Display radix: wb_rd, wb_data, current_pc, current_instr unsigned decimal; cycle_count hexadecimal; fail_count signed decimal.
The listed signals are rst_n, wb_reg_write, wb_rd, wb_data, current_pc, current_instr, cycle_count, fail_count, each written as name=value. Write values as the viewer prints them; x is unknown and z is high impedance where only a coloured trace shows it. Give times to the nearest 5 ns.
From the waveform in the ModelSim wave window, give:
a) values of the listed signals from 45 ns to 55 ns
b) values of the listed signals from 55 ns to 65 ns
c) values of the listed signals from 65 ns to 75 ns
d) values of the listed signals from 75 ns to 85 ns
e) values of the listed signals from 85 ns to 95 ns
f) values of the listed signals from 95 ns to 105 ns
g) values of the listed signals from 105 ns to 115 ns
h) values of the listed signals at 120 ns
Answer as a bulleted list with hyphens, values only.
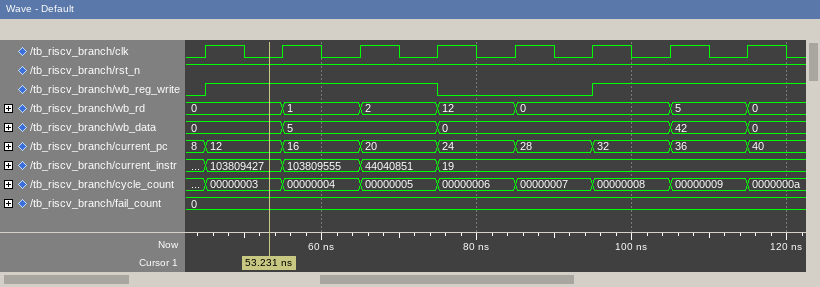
- rst_n=1, wb_reg_write=1, wb_rd=0, wb_data=0, current_pc=12, current_instr=103809427, cycle_count=00000003, fail_count=0
- rst_n=1, wb_reg_write=1, wb_rd=1, wb_data=5, current_pc=16, current_instr=103809555, cycle_count=00000004, fail_count=0
- rst_n=1, wb_reg_write=1, wb_rd=2, wb_data=5, current_pc=20, current_instr=44040851, cycle_count=00000005, fail_count=0
- rst_n=1, wb_reg_write=0, wb_rd=12, wb_data=0, current_pc=24, current_instr=19, cycle_count=00000006, fail_count=0
- rst_n=1, wb_reg_write=0, wb_rd=0, wb_data=0, current_pc=28, current_instr=19, cycle_count=00000007, fail_count=0
- rst_n=1, wb_reg_write=1, wb_rd=0, wb_data=0, current_pc=32, current_instr=19, cycle_count=00000008, fail_count=0
- rst_n=1, wb_reg_write=1, wb_rd=5, wb_data=42, current_pc=36, current_instr=19, cycle_count=00000009, fail_count=0
- rst_n=1, wb_reg_write=1, wb_rd=0, wb_data=0, current_pc=40, current_instr=19, cycle_count=0000000a, fail_count=0
